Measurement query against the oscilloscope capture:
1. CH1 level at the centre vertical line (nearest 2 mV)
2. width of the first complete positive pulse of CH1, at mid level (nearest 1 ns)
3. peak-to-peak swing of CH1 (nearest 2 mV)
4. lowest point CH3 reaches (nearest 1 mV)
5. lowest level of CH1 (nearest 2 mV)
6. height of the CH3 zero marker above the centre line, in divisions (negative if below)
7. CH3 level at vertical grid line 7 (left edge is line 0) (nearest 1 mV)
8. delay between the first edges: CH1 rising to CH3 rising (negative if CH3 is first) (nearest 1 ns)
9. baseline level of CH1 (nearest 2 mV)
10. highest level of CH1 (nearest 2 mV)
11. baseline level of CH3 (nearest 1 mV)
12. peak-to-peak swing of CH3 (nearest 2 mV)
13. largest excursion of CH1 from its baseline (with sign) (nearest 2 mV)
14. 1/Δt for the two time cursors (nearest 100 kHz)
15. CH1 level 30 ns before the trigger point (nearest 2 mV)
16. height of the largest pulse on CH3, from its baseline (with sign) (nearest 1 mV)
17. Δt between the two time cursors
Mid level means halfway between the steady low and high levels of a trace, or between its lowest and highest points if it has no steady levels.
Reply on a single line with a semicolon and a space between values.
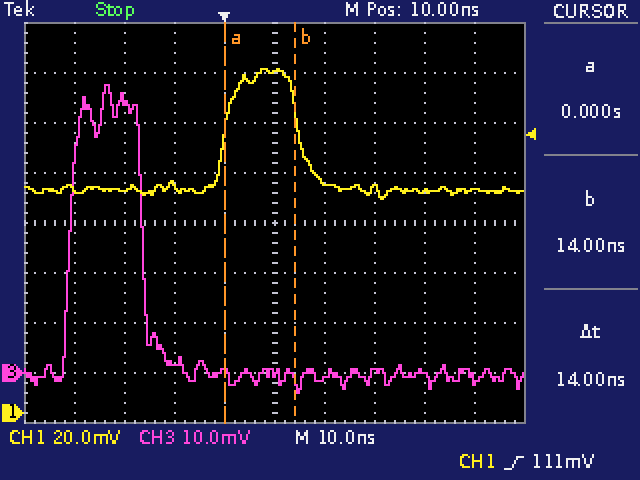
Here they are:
136 mV; 15 ns; 52 mV; -4 mV; 86 mV; -3.0 div; 0 mV; -31 ns; 90 mV; 138 mV; 0 mV; 62 mV; +48 mV; 71.4 MHz; 90 mV; +58 mV; 14 ns
